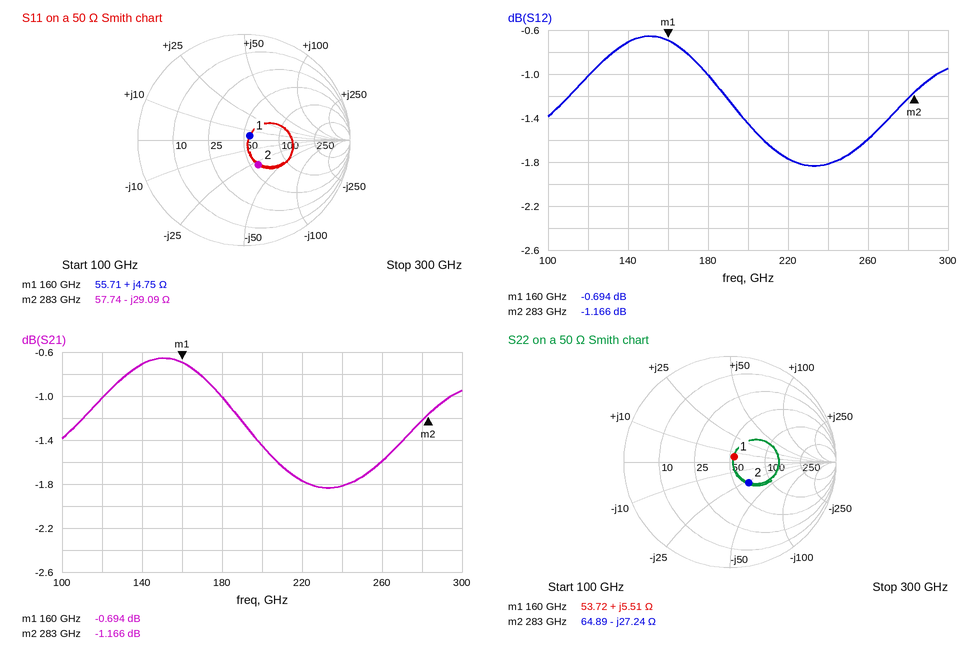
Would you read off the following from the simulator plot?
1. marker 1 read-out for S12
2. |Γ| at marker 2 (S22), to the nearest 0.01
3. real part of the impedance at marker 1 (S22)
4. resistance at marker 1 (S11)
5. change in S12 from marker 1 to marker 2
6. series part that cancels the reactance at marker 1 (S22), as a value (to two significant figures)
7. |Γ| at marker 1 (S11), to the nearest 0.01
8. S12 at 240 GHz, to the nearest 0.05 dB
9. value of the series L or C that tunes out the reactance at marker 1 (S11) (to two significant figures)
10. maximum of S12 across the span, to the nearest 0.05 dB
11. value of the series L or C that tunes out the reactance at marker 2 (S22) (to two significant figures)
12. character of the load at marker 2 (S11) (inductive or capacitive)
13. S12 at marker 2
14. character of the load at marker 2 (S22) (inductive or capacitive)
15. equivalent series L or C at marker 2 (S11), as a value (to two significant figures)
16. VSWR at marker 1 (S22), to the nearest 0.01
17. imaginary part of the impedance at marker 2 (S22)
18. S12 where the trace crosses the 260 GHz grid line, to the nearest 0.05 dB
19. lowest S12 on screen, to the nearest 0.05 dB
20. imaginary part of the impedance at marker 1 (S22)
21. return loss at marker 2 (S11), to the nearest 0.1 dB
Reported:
-0.694 dB
0.26
53.72 Ω
55.71 Ω
-0.472 dB
180 fF
0.07
-1.80 dB
210 fF
-0.65 dB
15 pH
capacitive
-1.166 dB
capacitive
19 fF
1.14
-27.24 Ω
-1.60 dB
-1.85 dB
+5.51 Ω
11.4 dB
